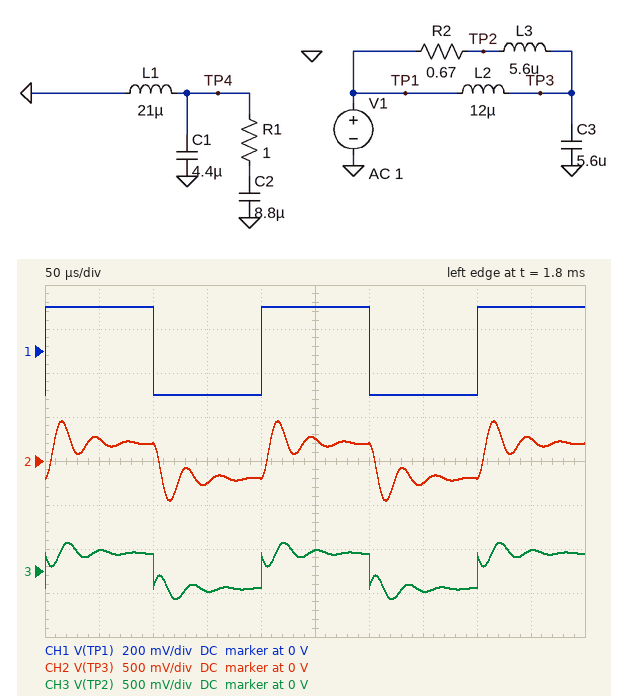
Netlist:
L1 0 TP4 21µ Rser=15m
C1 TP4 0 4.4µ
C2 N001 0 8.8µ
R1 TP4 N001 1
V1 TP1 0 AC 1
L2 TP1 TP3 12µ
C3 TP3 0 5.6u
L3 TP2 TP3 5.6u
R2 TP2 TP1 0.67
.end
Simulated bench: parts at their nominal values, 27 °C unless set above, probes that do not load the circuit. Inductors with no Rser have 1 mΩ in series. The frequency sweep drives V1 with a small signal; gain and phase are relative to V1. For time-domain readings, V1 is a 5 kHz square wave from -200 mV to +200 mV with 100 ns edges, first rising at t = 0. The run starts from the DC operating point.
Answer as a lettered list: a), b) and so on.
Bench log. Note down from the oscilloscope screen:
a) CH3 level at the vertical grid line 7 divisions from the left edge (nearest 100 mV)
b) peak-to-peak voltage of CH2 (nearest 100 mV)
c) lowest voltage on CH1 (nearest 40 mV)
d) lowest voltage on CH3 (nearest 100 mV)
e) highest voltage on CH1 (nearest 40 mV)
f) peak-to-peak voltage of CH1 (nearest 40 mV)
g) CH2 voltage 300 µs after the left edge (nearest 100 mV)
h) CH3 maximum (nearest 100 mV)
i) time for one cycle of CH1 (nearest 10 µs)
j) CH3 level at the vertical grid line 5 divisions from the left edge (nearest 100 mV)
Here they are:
a) -200 mV
b) 900 mV
c) -200 mV
d) -300 mV
e) 200 mV
f) 400 mV
g) 200 mV
h) 300 mV
i) 200 µs
j) 200 mV
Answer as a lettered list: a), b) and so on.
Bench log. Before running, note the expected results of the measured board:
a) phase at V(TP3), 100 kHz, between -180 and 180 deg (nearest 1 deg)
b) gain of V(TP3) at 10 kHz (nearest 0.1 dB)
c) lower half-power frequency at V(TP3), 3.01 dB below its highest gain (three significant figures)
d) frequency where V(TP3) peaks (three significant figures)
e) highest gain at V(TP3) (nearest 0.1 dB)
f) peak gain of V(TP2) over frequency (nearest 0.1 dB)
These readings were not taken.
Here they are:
a) -172 deg
b) 1.2 dB
c) 24.8 kHz
d) 32.0 kHz
e) 9.2 dB
f) 0.8 dB
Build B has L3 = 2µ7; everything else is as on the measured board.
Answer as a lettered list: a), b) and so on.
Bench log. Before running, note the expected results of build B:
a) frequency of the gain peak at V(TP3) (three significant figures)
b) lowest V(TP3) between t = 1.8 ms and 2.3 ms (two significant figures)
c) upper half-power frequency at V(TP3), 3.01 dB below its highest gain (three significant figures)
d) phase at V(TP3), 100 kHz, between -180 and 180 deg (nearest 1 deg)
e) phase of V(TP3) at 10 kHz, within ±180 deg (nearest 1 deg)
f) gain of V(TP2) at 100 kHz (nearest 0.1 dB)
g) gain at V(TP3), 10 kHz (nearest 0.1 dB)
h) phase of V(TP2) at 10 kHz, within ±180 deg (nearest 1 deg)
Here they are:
a) 36.2 kHz
b) -370 mV
c) 50.4 kHz
d) -159 deg
e) -7 deg
f) -0.9 dB
g) 1.1 dB
h) -8 deg
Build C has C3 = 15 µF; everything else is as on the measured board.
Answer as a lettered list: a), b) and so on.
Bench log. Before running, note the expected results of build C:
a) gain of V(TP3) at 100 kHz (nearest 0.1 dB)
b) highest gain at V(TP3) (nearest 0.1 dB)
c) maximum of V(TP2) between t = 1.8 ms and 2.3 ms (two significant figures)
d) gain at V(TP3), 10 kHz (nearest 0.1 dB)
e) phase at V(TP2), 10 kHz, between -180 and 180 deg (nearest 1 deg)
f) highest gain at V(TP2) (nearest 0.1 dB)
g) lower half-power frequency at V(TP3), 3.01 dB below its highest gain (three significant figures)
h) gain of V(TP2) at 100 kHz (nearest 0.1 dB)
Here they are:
a) -26.8 dB
b) 6.3 dB
c) 350 mV
d) 3.4 dB
e) -25 deg
f) 1.9 dB
g) 9.93 kHz
h) -0.2 dB
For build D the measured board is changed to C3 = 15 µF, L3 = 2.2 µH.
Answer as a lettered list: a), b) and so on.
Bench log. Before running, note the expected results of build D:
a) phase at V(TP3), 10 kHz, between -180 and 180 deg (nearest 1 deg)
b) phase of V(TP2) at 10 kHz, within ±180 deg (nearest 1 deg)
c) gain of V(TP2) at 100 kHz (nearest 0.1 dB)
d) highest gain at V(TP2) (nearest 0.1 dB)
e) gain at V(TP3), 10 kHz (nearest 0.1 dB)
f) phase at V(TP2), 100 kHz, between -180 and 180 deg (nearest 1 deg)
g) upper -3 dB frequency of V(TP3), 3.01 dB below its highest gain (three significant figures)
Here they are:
a) -23 deg
b) -26 deg
c) -1.1 dB
d) 2.1 dB
e) 2.7 dB
f) 28 deg
g) 24.4 kHz
